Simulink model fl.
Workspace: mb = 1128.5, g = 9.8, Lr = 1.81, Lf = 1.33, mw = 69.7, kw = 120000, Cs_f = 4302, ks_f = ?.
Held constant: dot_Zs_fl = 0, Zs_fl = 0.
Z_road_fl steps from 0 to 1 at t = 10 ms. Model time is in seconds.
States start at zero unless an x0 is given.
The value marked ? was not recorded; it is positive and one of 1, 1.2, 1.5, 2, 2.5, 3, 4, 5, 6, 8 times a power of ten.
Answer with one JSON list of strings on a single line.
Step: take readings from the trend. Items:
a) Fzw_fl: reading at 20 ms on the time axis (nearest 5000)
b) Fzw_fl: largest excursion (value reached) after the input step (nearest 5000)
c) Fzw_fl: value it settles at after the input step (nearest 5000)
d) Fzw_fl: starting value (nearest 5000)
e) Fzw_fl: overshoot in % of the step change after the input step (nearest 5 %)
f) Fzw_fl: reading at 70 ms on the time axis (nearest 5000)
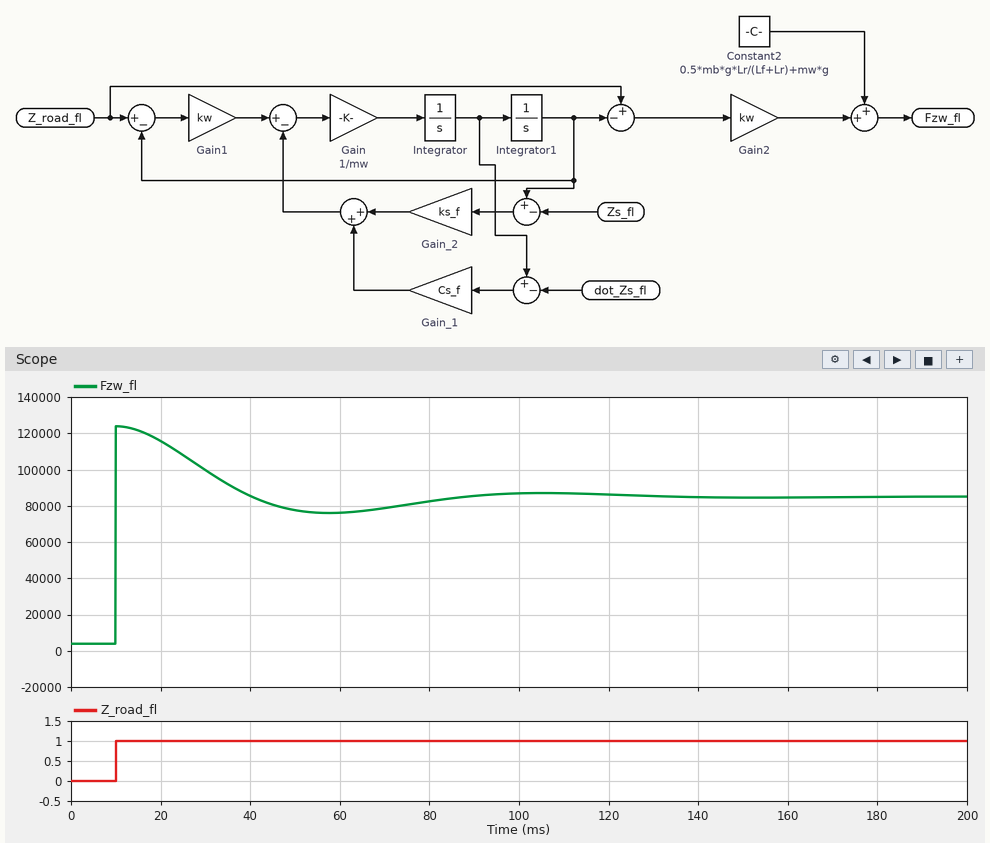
["115000", "125000", "85000", "5000", "50 %", "80000"]
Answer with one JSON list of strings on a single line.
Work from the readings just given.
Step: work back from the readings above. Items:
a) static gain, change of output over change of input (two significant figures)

["80000"]
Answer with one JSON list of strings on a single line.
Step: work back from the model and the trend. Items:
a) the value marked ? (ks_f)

["250000"]
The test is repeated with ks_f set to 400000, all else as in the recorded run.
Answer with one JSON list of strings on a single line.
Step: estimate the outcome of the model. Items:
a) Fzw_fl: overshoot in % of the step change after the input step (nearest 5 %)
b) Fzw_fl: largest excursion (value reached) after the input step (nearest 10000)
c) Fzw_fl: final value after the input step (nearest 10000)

["30 %", "120000", "100000"]
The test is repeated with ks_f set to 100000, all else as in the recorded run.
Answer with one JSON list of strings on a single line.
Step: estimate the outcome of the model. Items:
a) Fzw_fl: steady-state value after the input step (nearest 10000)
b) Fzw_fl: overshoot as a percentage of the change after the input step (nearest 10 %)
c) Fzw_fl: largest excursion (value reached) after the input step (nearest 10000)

["60000", "120 %", "120000"]
